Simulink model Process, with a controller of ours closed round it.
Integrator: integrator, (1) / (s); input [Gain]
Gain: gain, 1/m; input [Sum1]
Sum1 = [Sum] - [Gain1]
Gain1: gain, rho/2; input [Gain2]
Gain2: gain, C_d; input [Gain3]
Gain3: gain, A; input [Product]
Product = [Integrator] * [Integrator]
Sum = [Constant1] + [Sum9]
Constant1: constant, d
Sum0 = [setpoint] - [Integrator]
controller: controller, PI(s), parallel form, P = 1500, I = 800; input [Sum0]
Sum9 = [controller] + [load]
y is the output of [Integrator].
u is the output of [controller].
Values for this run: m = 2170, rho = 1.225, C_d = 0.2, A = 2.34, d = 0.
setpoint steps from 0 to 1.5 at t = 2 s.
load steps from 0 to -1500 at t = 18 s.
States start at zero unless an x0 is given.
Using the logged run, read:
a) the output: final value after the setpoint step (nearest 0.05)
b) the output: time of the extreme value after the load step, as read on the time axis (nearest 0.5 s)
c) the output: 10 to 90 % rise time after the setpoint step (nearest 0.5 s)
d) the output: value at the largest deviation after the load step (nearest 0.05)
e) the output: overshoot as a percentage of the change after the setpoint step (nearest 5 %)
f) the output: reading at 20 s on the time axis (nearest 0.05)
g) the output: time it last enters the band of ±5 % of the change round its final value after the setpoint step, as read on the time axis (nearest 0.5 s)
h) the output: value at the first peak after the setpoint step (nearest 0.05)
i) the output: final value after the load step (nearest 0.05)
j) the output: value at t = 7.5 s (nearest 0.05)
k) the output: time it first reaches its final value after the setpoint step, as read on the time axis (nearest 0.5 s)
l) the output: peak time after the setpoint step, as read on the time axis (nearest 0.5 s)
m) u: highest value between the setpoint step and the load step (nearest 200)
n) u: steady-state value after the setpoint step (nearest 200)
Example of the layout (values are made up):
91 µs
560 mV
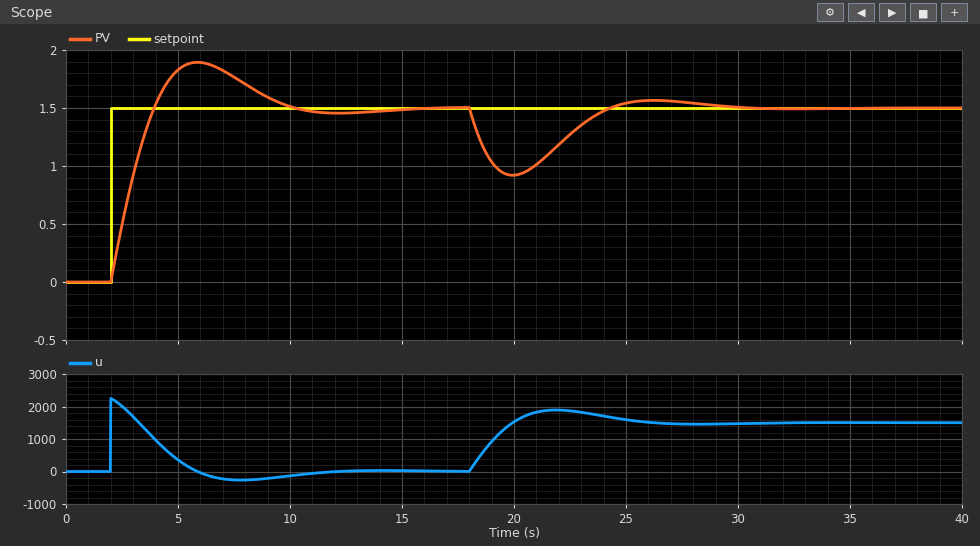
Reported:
1.50
20.0 s
1.5 s
0.90
25 %
0.90
9.0 s
1.90
1.50
1.75
4.0 s
6.0 s
2200
0
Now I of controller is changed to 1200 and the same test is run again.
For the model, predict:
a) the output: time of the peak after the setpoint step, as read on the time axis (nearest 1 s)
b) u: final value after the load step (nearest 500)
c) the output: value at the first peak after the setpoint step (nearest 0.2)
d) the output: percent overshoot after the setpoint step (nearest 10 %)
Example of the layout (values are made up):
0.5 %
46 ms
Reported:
5 s
1500
2.0
30 %
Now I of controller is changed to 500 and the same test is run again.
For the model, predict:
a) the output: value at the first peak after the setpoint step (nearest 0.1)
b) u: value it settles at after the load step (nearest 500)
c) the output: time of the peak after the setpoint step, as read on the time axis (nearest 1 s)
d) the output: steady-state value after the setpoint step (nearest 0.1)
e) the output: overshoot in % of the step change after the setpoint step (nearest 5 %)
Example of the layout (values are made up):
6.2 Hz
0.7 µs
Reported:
1.8
1500
7 s
1.5
20 %
